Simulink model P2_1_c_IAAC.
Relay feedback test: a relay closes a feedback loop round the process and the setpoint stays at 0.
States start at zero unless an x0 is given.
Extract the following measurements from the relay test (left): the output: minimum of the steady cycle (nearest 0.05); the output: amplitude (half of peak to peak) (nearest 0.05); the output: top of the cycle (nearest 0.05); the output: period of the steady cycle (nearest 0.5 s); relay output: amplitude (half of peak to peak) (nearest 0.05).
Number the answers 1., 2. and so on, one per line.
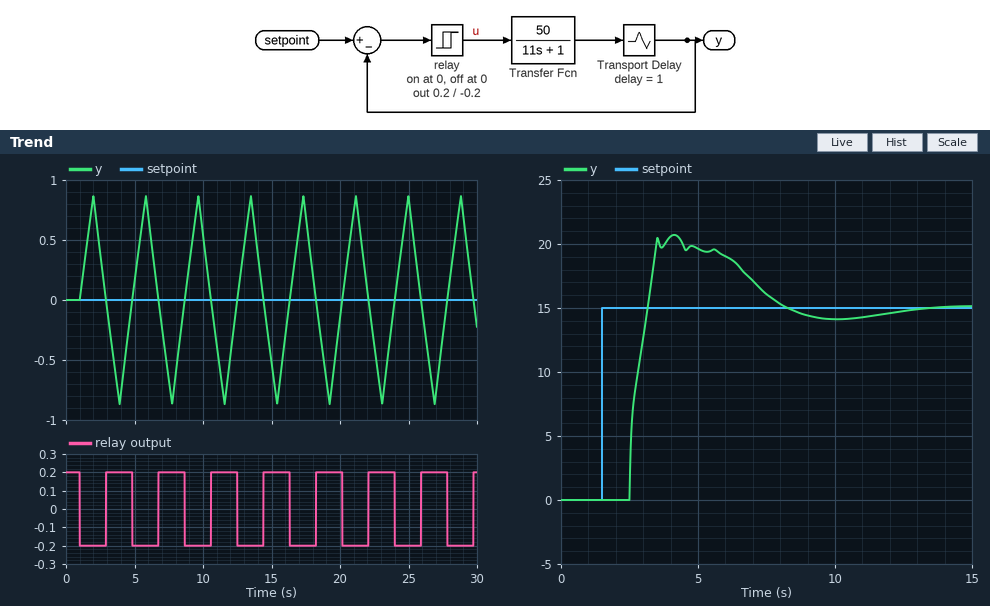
1. -0.85
2. 0.85
3. 0.85
4. 4.0 s
5. 0.20
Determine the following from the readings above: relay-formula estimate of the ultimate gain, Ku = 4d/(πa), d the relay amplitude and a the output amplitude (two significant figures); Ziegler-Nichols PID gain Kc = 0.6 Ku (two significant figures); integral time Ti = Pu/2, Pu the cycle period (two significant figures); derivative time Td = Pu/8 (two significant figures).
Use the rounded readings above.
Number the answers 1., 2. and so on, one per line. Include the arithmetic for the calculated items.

1. 4 × 0.2 / (π × 0.85) = 0.30
2. 0.6 × 0.3 = 0.18
3. 4 / 2 = 2.0 s
4. 4 / 8 = 0.50 s
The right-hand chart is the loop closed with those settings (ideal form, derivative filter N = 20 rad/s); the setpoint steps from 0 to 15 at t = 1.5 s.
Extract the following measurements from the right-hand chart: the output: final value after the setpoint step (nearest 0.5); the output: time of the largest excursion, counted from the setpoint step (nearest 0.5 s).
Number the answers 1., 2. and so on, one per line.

1. 15.0
2. 2.5 s
